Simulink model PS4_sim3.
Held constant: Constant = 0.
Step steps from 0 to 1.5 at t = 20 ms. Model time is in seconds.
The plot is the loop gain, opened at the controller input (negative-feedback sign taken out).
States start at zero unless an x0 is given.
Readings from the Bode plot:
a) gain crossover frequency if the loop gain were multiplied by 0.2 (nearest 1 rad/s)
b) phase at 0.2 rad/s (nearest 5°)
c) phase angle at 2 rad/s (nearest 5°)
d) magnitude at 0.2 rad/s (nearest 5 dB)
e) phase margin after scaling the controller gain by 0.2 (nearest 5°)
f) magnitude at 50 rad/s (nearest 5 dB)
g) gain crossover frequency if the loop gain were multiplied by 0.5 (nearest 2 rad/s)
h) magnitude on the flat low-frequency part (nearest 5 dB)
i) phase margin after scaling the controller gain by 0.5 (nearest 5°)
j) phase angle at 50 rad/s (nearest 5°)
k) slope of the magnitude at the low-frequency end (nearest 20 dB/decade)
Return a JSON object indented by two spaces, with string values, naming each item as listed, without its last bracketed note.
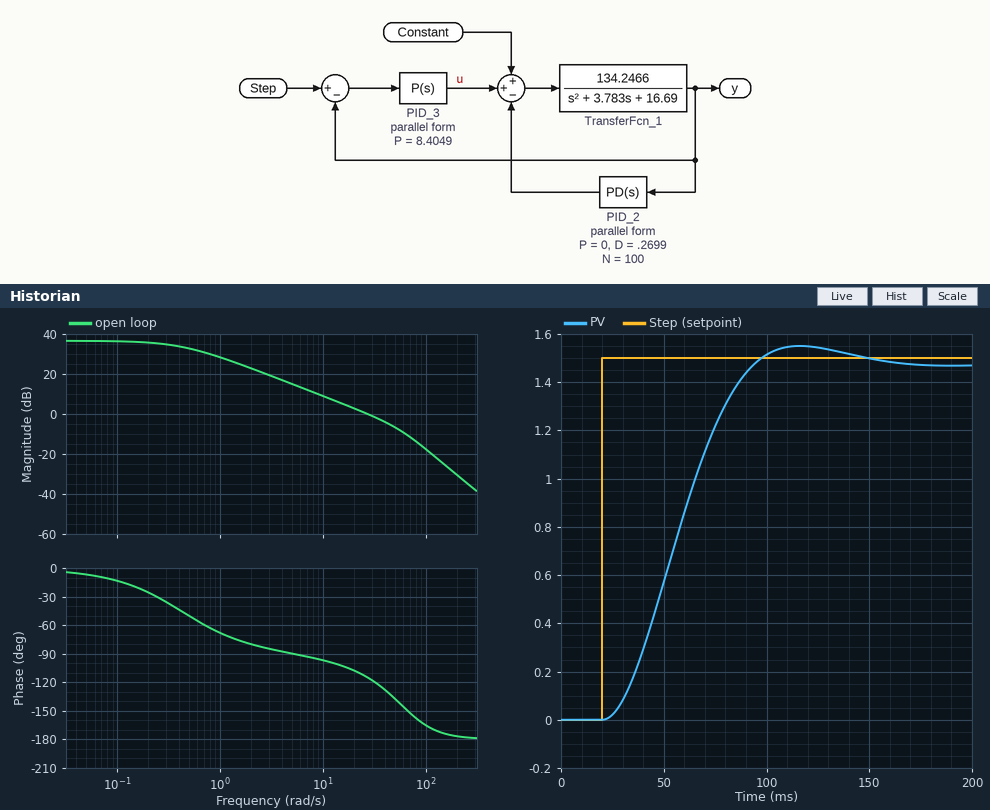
{
  "gain crossover frequency if the loop gain were multiplied by 0.2": "6 rad/s",
  "phase at 0.2 rad/s": "-25°",
  "phase angle at 2 rad/s": "-80°",
  "magnitude at 0.2 rad/s": "35 dB",
  "phase margin after scaling the controller gain by 0.2": "90°",
  "magnitude at 50 rad/s": "-5 dB",
  "gain crossover frequency if the loop gain were multiplied by 0.5": "14 rad/s",
  "magnitude on the flat low-frequency part": "35 dB",
  "phase margin after scaling the controller gain by 0.5": "80°",
  "phase angle at 50 rad/s": "-135°",
  "slope of the magnitude at the low-frequency end": "0 dB/decade"
}
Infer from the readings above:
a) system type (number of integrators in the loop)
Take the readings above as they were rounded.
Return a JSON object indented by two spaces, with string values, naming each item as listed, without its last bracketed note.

{
  "system type": "0"
}
